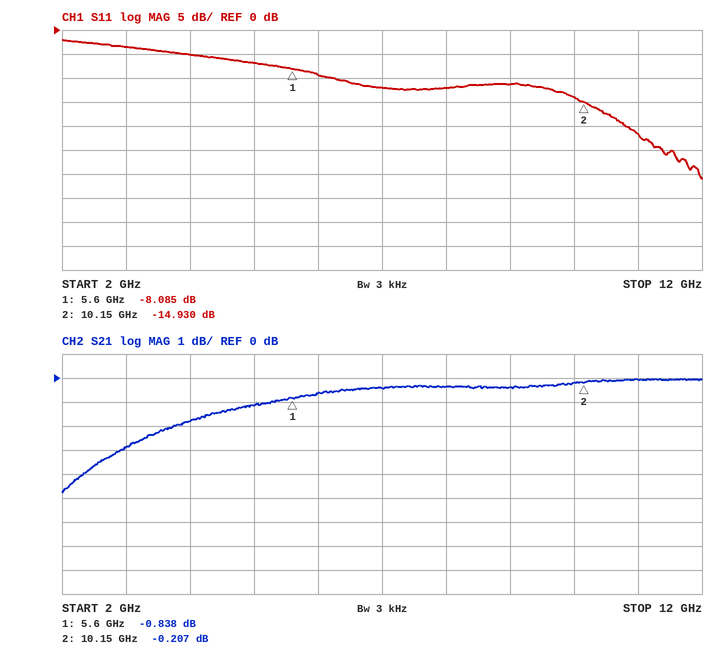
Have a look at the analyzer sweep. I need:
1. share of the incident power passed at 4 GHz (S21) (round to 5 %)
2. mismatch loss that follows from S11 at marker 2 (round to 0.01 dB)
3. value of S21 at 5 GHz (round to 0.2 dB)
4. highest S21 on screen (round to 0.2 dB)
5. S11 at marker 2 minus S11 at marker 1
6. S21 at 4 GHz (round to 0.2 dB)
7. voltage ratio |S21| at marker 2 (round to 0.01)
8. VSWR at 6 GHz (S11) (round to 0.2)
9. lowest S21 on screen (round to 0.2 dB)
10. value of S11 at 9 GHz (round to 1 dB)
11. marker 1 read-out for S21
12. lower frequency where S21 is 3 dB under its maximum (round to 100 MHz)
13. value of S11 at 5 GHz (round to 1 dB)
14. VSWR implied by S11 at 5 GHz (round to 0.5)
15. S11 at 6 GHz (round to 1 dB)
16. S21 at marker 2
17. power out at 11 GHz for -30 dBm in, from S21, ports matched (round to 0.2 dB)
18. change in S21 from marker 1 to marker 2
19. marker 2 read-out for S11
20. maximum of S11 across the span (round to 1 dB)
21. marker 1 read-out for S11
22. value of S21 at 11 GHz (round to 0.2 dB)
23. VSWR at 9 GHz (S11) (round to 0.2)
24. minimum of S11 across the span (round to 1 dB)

65 %
0.14 dB
-1.2 dB
0.0 dB
-6.845 dB
-1.8 dB
0.98
2.0
-4.8 dB
-11 dB
-0.838 dB
2.9 GHz
-7 dB
2.5
-9 dB
-0.207 dB
-30.0 dBm
0.631 dB
-14.930 dB
-2 dB
-8.085 dB
0.0 dB
1.8
-31 dB
